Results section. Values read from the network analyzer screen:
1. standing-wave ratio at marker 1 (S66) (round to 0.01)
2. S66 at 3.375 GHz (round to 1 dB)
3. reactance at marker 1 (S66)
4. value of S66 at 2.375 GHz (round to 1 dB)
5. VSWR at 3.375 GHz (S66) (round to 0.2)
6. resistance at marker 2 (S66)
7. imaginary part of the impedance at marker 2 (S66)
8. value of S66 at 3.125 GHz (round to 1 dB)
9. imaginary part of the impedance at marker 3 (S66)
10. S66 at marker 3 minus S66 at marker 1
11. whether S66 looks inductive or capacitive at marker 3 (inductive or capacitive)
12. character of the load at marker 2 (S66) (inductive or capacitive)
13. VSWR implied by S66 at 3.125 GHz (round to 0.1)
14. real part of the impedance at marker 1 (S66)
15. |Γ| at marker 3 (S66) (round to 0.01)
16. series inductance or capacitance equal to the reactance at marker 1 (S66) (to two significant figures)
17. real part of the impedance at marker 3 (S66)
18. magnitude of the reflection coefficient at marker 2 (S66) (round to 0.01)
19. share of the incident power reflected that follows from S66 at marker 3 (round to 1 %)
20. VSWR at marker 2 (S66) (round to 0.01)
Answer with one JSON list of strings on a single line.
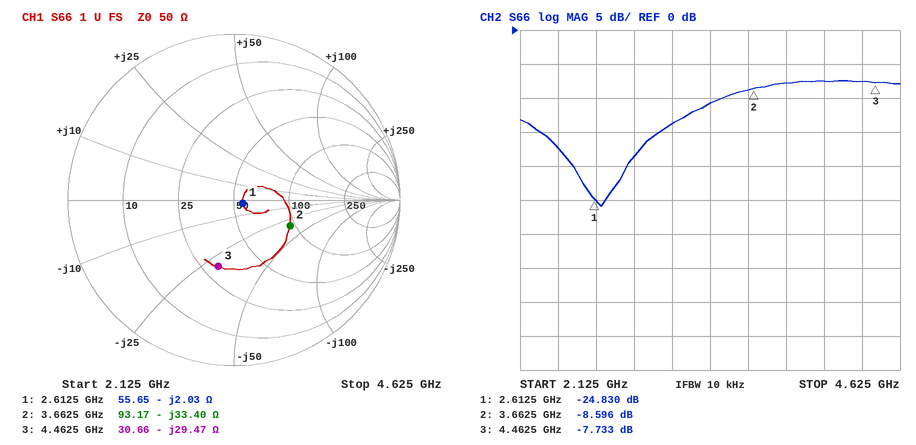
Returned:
["1.12", "-11 dB", "-2.03 Ω", "-17 dB", "1.8", "93.17 Ω", "-33.40 Ω", "-14 dB", "-29.47 Ω", "17.097 dB", "capacitive", "capacitive", "1.5", "55.65 Ω", "0.41", "30 pF", "30.66 Ω", "0.37", "17 %", "2.18"]
